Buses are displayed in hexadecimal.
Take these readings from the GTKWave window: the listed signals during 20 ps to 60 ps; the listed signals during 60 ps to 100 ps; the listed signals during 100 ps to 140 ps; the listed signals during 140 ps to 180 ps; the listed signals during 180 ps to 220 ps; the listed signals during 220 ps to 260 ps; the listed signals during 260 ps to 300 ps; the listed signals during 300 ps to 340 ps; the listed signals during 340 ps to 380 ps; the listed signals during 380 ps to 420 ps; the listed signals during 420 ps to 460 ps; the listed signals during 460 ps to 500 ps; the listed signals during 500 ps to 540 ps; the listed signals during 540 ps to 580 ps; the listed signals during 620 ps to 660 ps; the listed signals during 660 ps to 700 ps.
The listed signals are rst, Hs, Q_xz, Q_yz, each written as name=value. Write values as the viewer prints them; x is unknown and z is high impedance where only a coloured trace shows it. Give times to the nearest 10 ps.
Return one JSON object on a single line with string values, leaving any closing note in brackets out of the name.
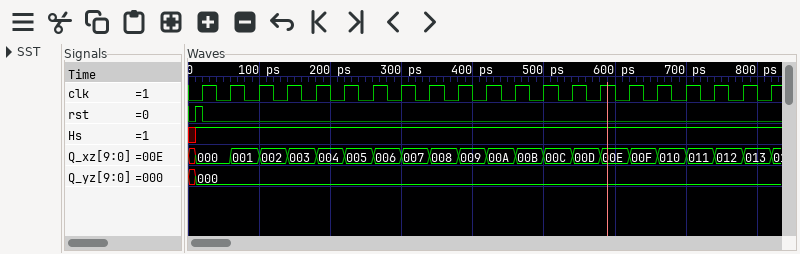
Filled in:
{"the listed signals during 20 ps to 60 ps": "rst=0, Hs=1, Q_xz=000, Q_yz=000", "the listed signals during 60 ps to 100 ps": "rst=0, Hs=1, Q_xz=001, Q_yz=000", "the listed signals during 100 ps to 140 ps": "rst=0, Hs=1, Q_xz=002, Q_yz=000", "the listed signals during 140 ps to 180 ps": "rst=0, Hs=1, Q_xz=003, Q_yz=000", "the listed signals during 180 ps to 220 ps": "rst=0, Hs=1, Q_xz=004, Q_yz=000", "the listed signals during 220 ps to 260 ps": "rst=0, Hs=1, Q_xz=005, Q_yz=000", "the listed signals during 260 ps to 300 ps": "rst=0, Hs=1, Q_xz=006, Q_yz=000", "the listed signals during 300 ps to 340 ps": "rst=0, Hs=1, Q_xz=007, Q_yz=000", "the listed signals during 340 ps to 380 ps": "rst=0, Hs=1, Q_xz=008, Q_yz=000", "the listed signals during 380 ps to 420 ps": "rst=0, Hs=1, Q_xz=009, Q_yz=000", "the listed signals during 420 ps to 460 ps": "rst=0, Hs=1, Q_xz=00A, Q_yz=000", "the listed signals during 460 ps to 500 ps": "rst=0, Hs=1, Q_xz=00B, Q_yz=000", "the listed signals during 500 ps to 540 ps": "rst=0, Hs=1, Q_xz=00C, Q_yz=000", "the listed signals during 540 ps to 580 ps": "rst=0, Hs=1, Q_xz=00D, Q_yz=000", "the listed signals during 620 ps to 660 ps": "rst=0, Hs=1, Q_xz=00F, Q_yz=000", "the listed signals during 660 ps to 700 ps": "rst=0, Hs=1, Q_xz=010, Q_yz=000"}
